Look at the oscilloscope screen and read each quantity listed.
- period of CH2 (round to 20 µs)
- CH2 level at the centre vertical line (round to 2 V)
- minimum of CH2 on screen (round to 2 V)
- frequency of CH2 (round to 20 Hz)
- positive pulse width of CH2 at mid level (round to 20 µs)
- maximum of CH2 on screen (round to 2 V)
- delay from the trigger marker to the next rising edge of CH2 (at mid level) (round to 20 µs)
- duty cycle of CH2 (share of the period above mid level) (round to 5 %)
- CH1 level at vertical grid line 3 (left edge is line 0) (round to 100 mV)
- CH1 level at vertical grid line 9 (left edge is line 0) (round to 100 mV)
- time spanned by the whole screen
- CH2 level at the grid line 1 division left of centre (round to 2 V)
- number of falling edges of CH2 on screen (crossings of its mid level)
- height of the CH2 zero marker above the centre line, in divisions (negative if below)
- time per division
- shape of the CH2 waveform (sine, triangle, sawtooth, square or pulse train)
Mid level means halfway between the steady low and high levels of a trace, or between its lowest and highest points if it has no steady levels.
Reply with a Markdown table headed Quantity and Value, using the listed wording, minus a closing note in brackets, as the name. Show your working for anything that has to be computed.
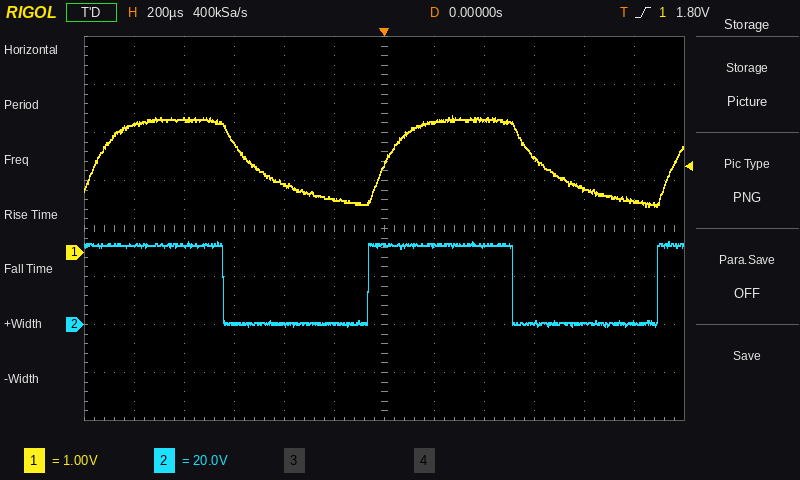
| Quantity | Value |
|---|---|
| period of CH2 | 1.16 ms |
| CH2 level at the centre vertical line | 34 V |
| minimum of CH2 on screen | 0 V |
| frequency of CH2 | 1 / 1.16 ms ≈ 862 Hz, so 860 Hz to the nearest 20 Hz |
| positive pulse width of CH2 at mid level | 580 µs |
| maximum of CH2 on screen | 34 V |
| delay from the trigger marker to the next rising edge of CH2 (at mid level) | 1.10 ms |
| duty cycle of CH2 (share of the period above mid level) | 580 µs / 1.16 ms ≈ 50 % |
| CH1 level at vertical grid line 3 (left edge is line 0) | 2.3 V |
| CH1 level at vertical grid line 9 (left edge is line 0) | 2.0 V |
| time spanned by the whole screen | 2.4 ms |
| CH2 level at the grid line 1 division left of centre | 0 V |
| number of falling edges of CH2 on screen | 2 |
| height of the CH2 zero marker above the centre line, in divisions | -2.0 div |
| time per division | 200 µs |
| shape of the CH2 waveform | square |
